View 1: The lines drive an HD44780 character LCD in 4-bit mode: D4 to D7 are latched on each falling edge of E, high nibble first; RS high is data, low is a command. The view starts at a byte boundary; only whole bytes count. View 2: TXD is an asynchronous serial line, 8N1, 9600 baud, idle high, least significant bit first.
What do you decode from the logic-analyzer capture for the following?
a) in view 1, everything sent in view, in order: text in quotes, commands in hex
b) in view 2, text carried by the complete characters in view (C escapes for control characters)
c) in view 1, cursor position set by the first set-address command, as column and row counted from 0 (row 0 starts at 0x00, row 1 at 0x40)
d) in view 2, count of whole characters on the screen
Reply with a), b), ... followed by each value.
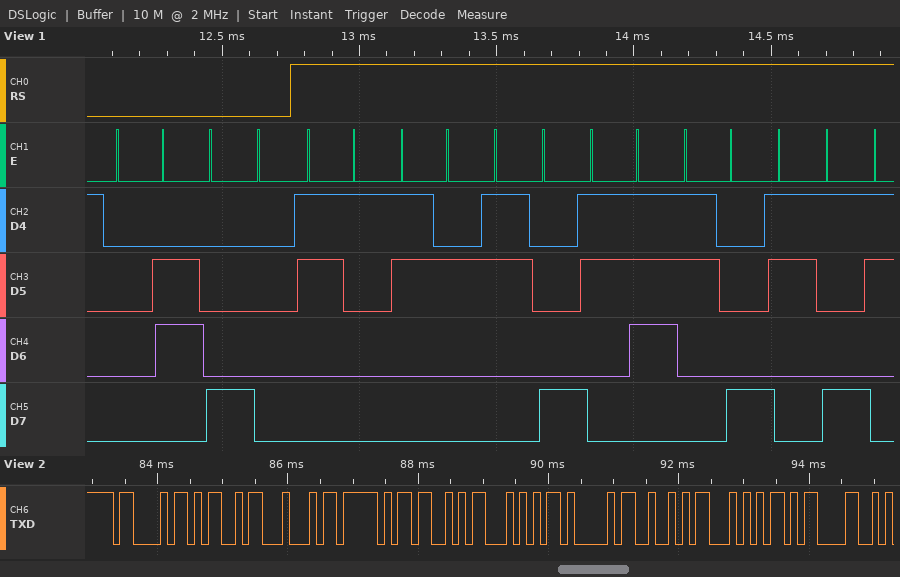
a) 0x06 0x80 "128789"
b) "CMD_START\r"
c) column 0, row 0
d) 10
